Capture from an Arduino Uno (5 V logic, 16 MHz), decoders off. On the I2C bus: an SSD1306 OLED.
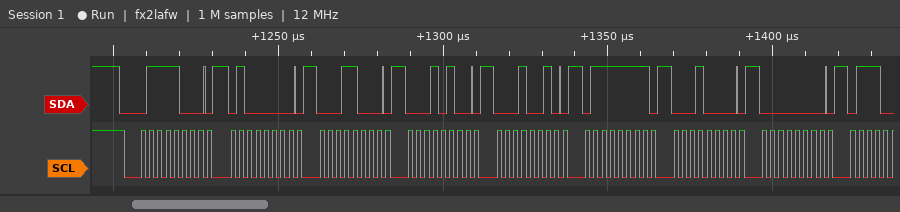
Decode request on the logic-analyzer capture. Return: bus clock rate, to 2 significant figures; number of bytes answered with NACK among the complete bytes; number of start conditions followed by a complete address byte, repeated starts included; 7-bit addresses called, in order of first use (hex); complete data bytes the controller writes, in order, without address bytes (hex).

400 kHz
0
1
0x3C
40 18 14 12 7F 10 00
